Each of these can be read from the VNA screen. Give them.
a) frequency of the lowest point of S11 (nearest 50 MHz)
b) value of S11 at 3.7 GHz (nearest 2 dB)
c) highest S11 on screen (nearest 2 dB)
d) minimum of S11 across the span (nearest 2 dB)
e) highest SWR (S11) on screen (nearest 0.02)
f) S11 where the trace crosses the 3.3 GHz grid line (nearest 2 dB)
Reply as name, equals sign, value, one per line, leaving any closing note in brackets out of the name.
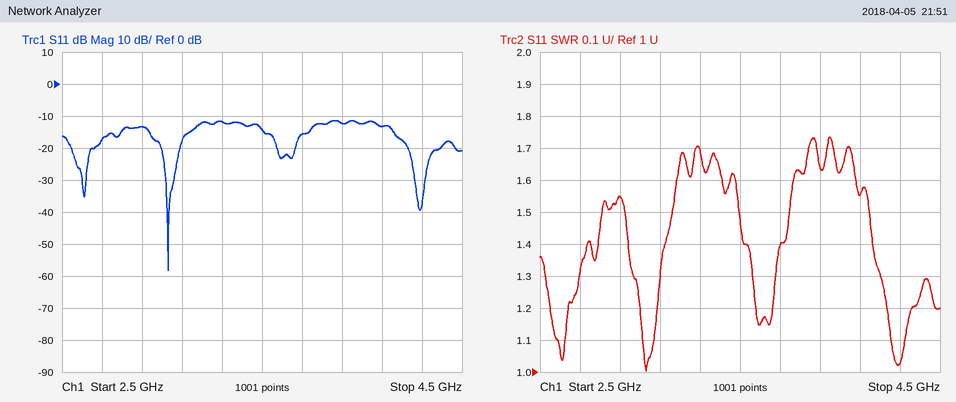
frequency of the lowest point of S11 = 3.05 GHz
value of S11 at 3.7 GHz = -16 dB
highest S11 on screen = -12 dB
minimum of S11 across the span = -58 dB
highest SWR (S11) on screen = 1.74
S11 where the trace crosses the 3.3 GHz grid line = -12 dB
